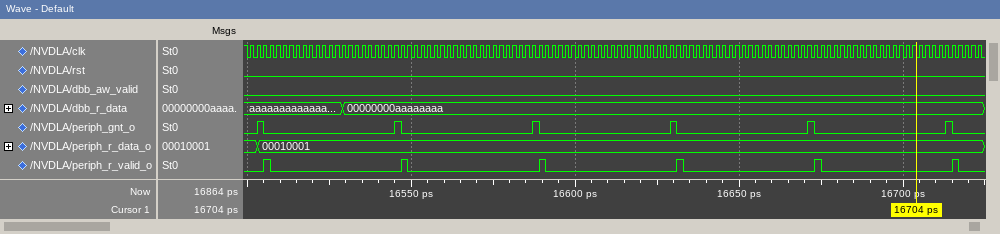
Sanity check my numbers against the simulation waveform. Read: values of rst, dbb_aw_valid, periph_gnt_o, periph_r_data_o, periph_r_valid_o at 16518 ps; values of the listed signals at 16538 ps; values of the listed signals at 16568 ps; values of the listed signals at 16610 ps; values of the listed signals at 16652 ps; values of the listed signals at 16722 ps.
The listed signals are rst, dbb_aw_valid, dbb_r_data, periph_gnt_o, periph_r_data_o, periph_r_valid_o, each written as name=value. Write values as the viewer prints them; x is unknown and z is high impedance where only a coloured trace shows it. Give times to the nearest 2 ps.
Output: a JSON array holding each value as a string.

["rst=0, dbb_aw_valid=0, periph_gnt_o=0, periph_r_data_o=00010001, periph_r_valid_o=0", "rst=0, dbb_aw_valid=0, dbb_r_data=00000000aaaaaaaa, periph_gnt_o=0, periph_r_data_o=00010001, periph_r_valid_o=0", "rst=0, dbb_aw_valid=0, dbb_r_data=00000000aaaaaaaa, periph_gnt_o=0, periph_r_data_o=00010001, periph_r_valid_o=0", "rst=0, dbb_aw_valid=0, dbb_r_data=00000000aaaaaaaa, periph_gnt_o=0, periph_r_data_o=00010001, periph_r_valid_o=0", "rst=0, dbb_aw_valid=0, dbb_r_data=00000000aaaaaaaa, periph_gnt_o=0, periph_r_data_o=00010001, periph_r_valid_o=0", "rst=0, dbb_aw_valid=0, dbb_r_data=00000000aaaaaaaa, periph_gnt_o=0, periph_r_data_o=00010001, periph_r_valid_o=0"]
